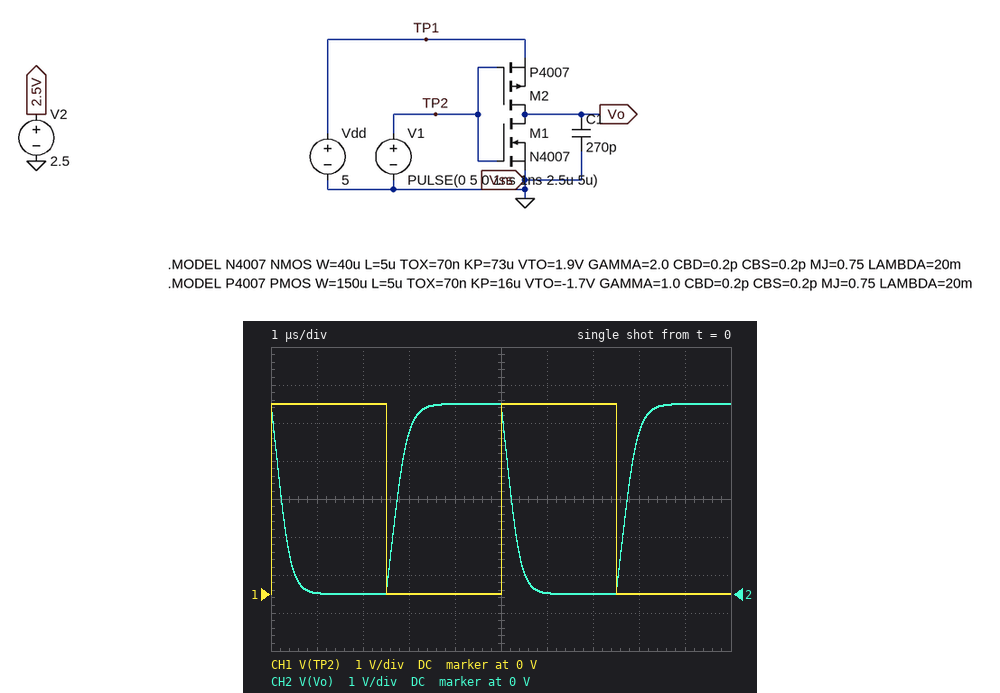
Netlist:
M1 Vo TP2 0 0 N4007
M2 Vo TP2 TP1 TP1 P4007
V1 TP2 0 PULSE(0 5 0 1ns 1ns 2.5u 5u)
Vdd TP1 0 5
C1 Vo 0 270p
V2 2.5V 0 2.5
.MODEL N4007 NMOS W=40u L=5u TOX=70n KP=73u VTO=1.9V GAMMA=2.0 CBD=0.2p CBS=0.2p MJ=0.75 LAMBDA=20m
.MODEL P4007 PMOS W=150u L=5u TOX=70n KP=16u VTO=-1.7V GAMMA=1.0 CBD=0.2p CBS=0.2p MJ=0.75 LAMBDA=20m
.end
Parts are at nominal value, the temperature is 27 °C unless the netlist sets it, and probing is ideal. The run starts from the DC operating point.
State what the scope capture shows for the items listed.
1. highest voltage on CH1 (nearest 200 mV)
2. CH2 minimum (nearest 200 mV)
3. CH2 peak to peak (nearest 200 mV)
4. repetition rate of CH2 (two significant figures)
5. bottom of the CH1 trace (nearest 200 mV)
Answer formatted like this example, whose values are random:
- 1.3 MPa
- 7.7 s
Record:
- 5.0 V
- 0 V
- 5.0 V
- 200 kHz
- 0 V
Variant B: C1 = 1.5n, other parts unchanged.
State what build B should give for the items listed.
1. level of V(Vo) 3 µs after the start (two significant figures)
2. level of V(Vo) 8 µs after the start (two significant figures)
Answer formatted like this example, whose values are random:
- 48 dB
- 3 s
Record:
- 1.7 V
- 1.5 V
